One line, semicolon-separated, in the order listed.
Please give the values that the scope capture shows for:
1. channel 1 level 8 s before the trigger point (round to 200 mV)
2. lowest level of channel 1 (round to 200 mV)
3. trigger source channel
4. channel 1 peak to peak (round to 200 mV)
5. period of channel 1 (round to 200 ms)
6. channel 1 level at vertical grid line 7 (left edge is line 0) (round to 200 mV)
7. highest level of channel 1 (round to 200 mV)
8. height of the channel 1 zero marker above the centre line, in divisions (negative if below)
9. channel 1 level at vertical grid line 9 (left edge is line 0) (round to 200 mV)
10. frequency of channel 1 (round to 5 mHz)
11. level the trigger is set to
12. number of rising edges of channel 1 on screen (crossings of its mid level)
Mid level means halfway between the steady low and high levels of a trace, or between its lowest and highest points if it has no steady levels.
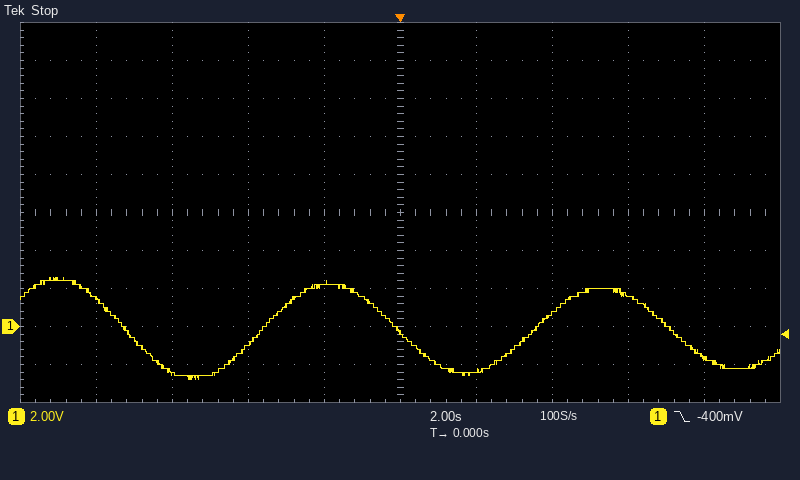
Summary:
1.4 V; -2.8 V; channel 1; 5.4 V; 7.2 s; 600 mV; 2.6 V; -3.0 div; -1.6 V; 140 mHz; -400 mV; 2
